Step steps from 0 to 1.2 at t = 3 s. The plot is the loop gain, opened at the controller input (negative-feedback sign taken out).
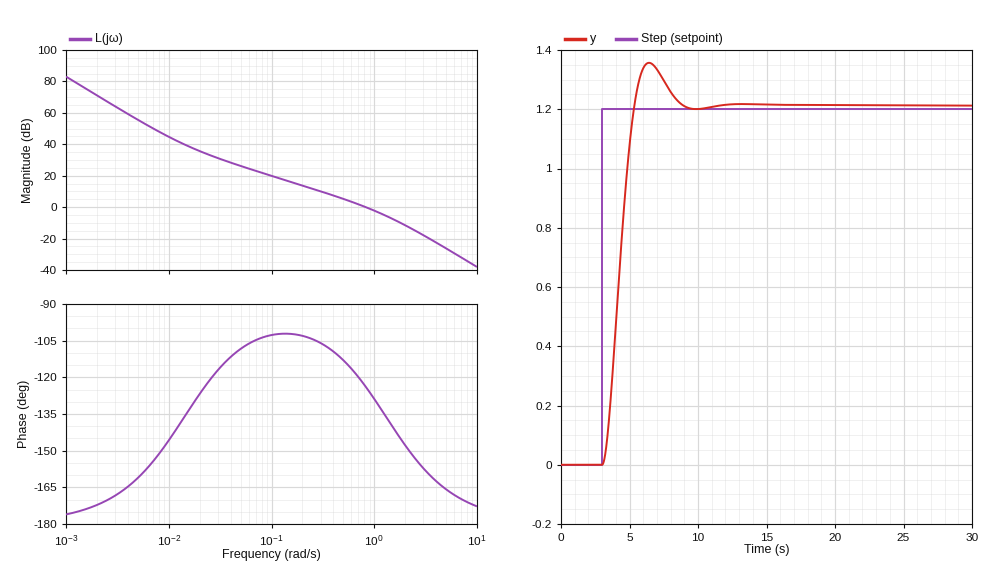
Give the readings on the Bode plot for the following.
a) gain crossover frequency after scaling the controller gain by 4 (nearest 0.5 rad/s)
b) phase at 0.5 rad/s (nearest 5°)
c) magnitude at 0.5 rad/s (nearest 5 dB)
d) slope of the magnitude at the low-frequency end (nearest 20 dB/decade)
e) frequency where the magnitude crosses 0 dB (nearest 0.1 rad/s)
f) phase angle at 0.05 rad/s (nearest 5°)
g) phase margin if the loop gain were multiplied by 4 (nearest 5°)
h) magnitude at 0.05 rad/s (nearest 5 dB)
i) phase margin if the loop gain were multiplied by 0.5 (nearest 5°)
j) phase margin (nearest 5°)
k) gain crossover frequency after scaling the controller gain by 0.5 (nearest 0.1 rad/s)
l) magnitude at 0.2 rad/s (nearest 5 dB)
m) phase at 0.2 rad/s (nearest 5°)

2.0 rad/s
-115°
5 dB
-40 dB/decade
0.8 rad/s
-110°
30°
25 dB
70°
55°
0.5 rad/s
15 dB
-105°
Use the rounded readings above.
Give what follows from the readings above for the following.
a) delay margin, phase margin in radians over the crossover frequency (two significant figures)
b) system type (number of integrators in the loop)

1.2 s
2
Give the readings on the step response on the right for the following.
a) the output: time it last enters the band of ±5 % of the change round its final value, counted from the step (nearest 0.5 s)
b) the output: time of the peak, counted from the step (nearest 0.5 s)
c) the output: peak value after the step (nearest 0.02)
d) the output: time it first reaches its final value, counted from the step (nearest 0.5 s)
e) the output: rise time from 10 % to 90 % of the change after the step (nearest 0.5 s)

5.0 s
3.5 s
1.36
2.5 s
1.5 s
